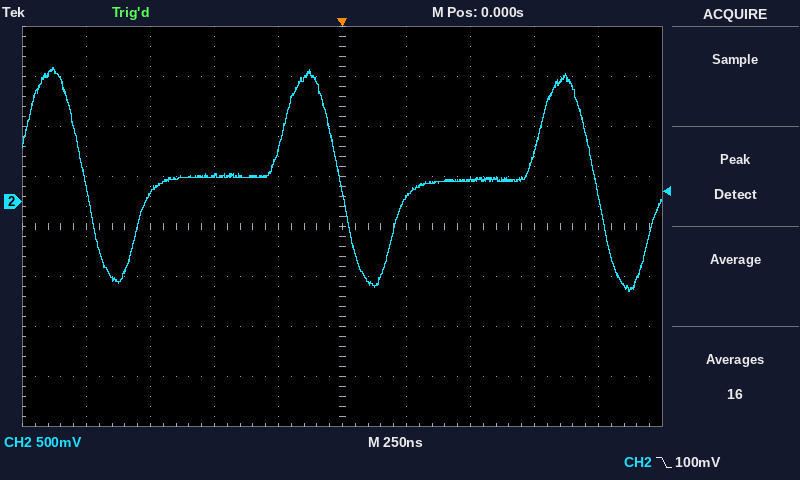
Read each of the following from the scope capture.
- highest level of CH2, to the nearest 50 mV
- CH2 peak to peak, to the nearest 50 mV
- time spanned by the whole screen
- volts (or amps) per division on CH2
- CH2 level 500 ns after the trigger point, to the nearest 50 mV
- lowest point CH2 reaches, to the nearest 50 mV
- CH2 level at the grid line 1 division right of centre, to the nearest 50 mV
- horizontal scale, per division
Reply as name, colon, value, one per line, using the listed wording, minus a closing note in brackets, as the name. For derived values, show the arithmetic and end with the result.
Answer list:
highest level of CH2, to the nearest 50 mV: 1.35 V
CH2 peak to peak, to the nearest 50 mV: 1.35 V − (-900 mV) = 2.25 V
time spanned by the whole screen: 2.5 µs
volts (or amps) per division on CH2: 500 mV
CH2 level 500 ns after the trigger point, to the nearest 50 mV: 200 mV
lowest point CH2 reaches, to the nearest 50 mV: -900 mV
CH2 level at the grid line 1 division right of centre, to the nearest 50 mV: 50 mV
horizontal scale, per division: 250 ns
